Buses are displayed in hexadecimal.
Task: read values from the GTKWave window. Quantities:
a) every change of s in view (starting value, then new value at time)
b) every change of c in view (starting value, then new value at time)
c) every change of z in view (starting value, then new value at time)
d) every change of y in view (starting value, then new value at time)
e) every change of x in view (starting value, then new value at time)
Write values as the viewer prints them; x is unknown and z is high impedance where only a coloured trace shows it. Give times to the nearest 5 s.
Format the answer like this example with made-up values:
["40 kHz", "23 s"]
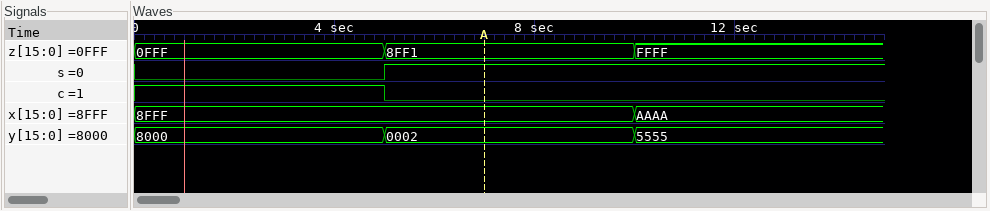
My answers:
["0, 1 at 5 s", "1, 0 at 5 s", "0FFF, 8FF1 at 5 s, FFFF at 10 s", "8000, 0002 at 5 s, 5555 at 10 s", "8FFF, AAAA at 10 s"]
